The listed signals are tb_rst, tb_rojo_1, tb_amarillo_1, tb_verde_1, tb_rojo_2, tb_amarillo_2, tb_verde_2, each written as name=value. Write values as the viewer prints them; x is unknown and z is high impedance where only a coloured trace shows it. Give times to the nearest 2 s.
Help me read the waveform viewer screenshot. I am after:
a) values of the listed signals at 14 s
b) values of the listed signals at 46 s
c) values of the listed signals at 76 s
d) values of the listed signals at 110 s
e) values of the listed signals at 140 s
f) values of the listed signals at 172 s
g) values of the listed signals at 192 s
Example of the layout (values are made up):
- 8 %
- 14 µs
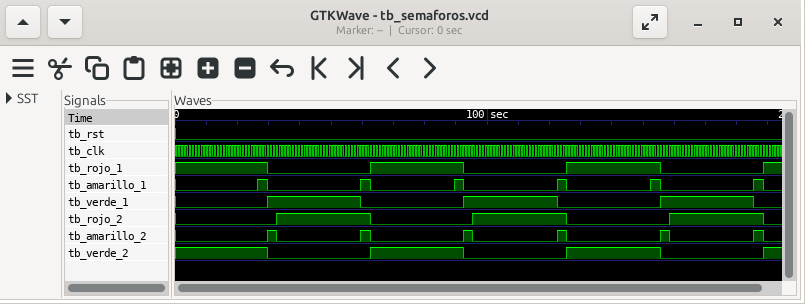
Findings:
- tb_rst=0, tb_rojo_1=1, tb_amarillo_1=0, tb_verde_1=0, tb_rojo_2=0, tb_amarillo_2=0, tb_verde_2=1
- tb_rst=0, tb_rojo_1=0, tb_amarillo_1=0, tb_verde_1=1, tb_rojo_2=1, tb_amarillo_2=0, tb_verde_2=0
- tb_rst=0, tb_rojo_1=1, tb_amarillo_1=0, tb_verde_1=0, tb_rojo_2=0, tb_amarillo_2=0, tb_verde_2=1
- tb_rst=0, tb_rojo_1=0, tb_amarillo_1=0, tb_verde_1=1, tb_rojo_2=1, tb_amarillo_2=0, tb_verde_2=0
- tb_rst=0, tb_rojo_1=1, tb_amarillo_1=0, tb_verde_1=0, tb_rojo_2=0, tb_amarillo_2=0, tb_verde_2=1
- tb_rst=0, tb_rojo_1=0, tb_amarillo_1=0, tb_verde_1=1, tb_rojo_2=1, tb_amarillo_2=0, tb_verde_2=0
- tb_rst=0, tb_rojo_1=1, tb_amarillo_1=0, tb_verde_1=0, tb_rojo_2=0, tb_amarillo_2=0, tb_verde_2=1
